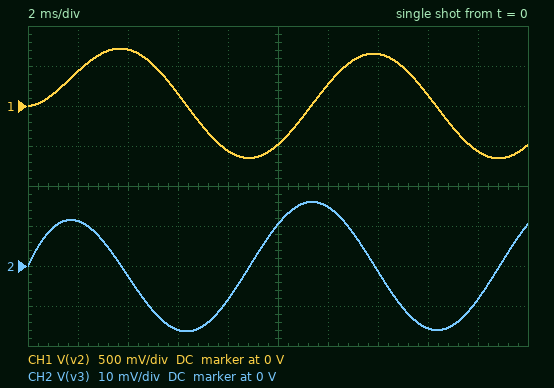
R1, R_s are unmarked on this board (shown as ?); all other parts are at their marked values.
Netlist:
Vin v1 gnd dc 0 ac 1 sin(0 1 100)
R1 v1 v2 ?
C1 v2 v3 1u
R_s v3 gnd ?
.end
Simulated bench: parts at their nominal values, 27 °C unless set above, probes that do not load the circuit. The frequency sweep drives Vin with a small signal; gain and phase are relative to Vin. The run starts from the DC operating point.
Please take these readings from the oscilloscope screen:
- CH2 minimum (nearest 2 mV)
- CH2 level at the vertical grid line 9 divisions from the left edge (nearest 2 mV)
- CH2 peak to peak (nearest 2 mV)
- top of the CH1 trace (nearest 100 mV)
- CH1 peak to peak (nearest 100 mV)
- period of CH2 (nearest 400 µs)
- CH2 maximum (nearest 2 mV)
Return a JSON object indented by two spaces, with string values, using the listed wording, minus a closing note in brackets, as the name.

{
  "CH2 minimum": "-16 mV",
  "CH2 level at the vertical grid line 9 divisions from the left edge": "-8 mV",
  "CH2 peak to peak": "32 mV",
  "top of the CH1 trace": "700 mV",
  "CH1 peak to peak": "1.4 V",
  "period of CH2": "10.0 ms",
  "CH2 maximum": "16 mV"
}
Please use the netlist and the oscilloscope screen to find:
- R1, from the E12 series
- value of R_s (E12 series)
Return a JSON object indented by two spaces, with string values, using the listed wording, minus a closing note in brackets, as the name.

{
  "R1, from the E12 series": "1.8 kΩ",
  "value of R_s": "39 Ω"
}
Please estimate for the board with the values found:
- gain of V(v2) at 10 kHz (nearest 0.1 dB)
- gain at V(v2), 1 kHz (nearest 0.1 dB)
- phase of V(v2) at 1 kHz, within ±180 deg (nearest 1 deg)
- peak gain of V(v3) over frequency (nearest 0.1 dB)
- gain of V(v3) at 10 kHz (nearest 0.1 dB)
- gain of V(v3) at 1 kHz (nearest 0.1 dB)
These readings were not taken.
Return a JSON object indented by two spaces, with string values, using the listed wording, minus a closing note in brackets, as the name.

{
  "gain of V(v2) at 10 kHz": "-32.8 dB",
  "gain at V(v2), 1 kHz": "-21.0 dB",
  "phase of V(v2) at 1 kHz, within ±180 deg": "-71 deg",
  "peak gain of V(v3) over frequency": "-33.5 dB",
  "gain of V(v3) at 10 kHz": "-33.5 dB",
  "gain of V(v3) at 1 kHz": "-33.5 dB"
}
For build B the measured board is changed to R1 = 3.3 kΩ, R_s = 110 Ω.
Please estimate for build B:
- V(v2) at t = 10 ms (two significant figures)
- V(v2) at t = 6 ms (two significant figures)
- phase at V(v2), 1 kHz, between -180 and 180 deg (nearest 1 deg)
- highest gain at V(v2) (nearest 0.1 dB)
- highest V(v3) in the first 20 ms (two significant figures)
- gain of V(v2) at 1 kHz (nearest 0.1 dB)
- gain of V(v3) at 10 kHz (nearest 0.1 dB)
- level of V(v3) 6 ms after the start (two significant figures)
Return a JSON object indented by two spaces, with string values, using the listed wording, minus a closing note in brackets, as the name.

{
  "V(v2) at t = 10 ms": "-350 mV",
  "V(v2) at t = 6 ms": "240 mV",
  "phase at V(v2), 1 kHz, between -180 and 180 deg": "-53 deg",
  "highest gain at V(v2)": "0 dB",
  "highest V(v3) in the first 20 ms": "29 mV",
  "gain of V(v2) at 1 kHz": "-24.9 dB",
  "gain of V(v3) at 10 kHz": "-29.8 dB",
  "level of V(v3) 6 ms after the start": "-28 mV"
}
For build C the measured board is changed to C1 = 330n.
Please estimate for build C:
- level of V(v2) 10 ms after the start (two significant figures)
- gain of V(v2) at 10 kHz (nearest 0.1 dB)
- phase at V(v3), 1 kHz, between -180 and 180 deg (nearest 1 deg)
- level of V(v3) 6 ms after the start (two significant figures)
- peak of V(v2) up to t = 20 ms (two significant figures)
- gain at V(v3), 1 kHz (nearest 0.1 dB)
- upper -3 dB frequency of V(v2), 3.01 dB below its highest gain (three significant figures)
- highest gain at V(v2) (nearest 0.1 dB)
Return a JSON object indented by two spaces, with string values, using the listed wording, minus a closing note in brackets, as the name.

{
  "level of V(v2) 10 ms after the start": "-330 mV",
  "gain of V(v2) at 10 kHz": "-29.4 dB",
  "phase at V(v3), 1 kHz, between -180 and 180 deg": "15 deg",
  "level of V(v3) 6 ms after the start": "-7.3 mV",
  "peak of V(v2) up to t = 20 ms": "940 mV",
  "gain at V(v3), 1 kHz": "-33.8 dB",
  "upper -3 dB frequency of V(v2), 3.01 dB below its highest gain": "262 Hz",
  "highest gain at V(v2)": "0 dB"
}
